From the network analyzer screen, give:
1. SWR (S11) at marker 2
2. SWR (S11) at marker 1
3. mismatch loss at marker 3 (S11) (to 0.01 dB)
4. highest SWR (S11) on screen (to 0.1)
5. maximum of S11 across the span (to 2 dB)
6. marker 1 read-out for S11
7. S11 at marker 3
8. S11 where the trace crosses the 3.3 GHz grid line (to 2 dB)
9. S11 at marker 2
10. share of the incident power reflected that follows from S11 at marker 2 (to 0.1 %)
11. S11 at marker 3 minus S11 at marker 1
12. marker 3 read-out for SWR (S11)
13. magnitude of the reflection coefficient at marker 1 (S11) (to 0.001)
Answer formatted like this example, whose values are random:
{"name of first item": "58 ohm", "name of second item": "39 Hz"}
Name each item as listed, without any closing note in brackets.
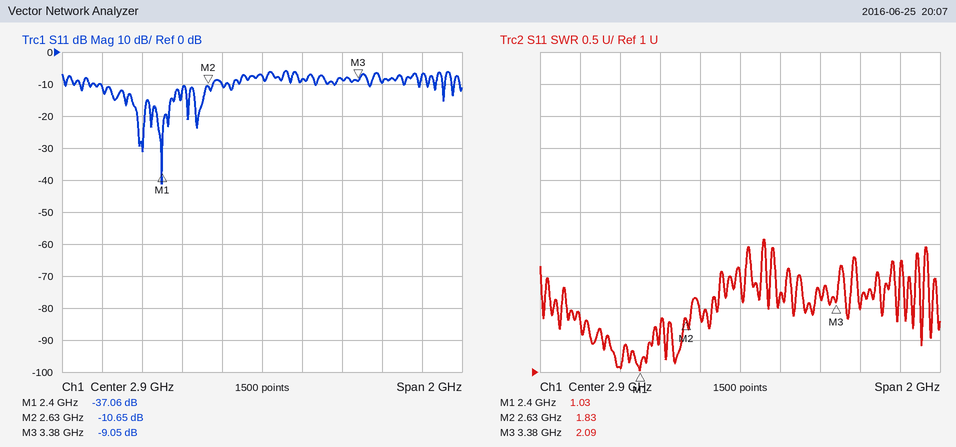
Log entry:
{"SWR (S11) at marker 2": "1.83", "SWR (S11) at marker 1": "1.03", "mismatch loss at marker 3 (S11)": "0.58 dB", "highest SWR (S11) on screen": "3.1", "maximum of S11 across the span": "-6 dB", "marker 1 read-out for S11": "-37.06 dB", "S11 at marker 3": "-9.05 dB", "S11 where the trace crosses the 3.3 GHz grid line": "-8 dB", "S11 at marker 2": "-10.65 dB", "share of the incident power reflected that follows from S11 at marker 2": "8.6 %", "S11 at marker 3 minus S11 at marker 1": "28.01 dB", "marker 3 read-out for SWR": "2.09", "magnitude of the reflection coefficient at marker 1 (S11)": "0.014"}
